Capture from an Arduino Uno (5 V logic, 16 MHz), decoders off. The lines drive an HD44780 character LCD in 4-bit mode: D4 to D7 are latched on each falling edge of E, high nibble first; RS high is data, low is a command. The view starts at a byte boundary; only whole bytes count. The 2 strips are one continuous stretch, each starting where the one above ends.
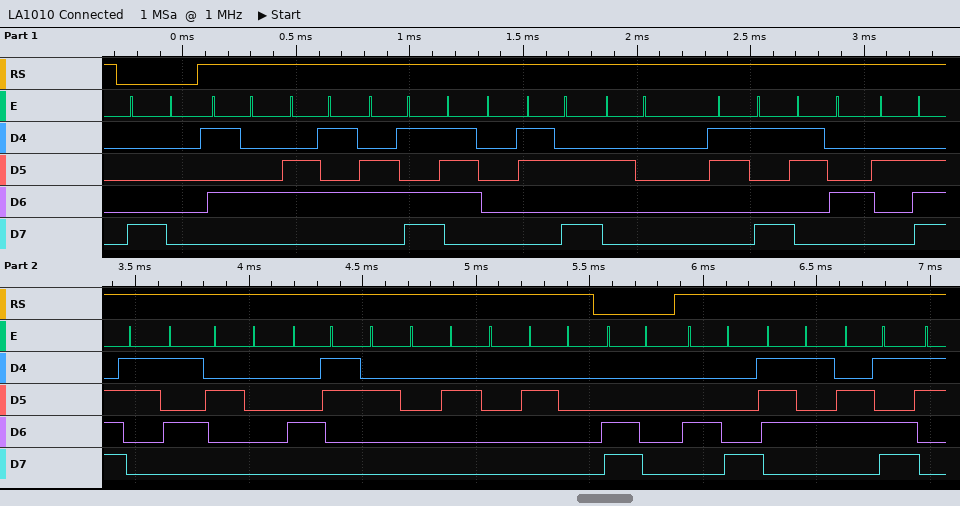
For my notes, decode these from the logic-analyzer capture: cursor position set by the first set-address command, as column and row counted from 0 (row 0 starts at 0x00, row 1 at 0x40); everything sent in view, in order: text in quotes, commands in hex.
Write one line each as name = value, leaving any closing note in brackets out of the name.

cursor position set by the first set-address command, as column and row counted from 0 = column 0, row 0
everything sent in view, in order: text in quotes, commands in hex = 0x80 "Temp: 94.5 C   " 0xC0 "Hum"
